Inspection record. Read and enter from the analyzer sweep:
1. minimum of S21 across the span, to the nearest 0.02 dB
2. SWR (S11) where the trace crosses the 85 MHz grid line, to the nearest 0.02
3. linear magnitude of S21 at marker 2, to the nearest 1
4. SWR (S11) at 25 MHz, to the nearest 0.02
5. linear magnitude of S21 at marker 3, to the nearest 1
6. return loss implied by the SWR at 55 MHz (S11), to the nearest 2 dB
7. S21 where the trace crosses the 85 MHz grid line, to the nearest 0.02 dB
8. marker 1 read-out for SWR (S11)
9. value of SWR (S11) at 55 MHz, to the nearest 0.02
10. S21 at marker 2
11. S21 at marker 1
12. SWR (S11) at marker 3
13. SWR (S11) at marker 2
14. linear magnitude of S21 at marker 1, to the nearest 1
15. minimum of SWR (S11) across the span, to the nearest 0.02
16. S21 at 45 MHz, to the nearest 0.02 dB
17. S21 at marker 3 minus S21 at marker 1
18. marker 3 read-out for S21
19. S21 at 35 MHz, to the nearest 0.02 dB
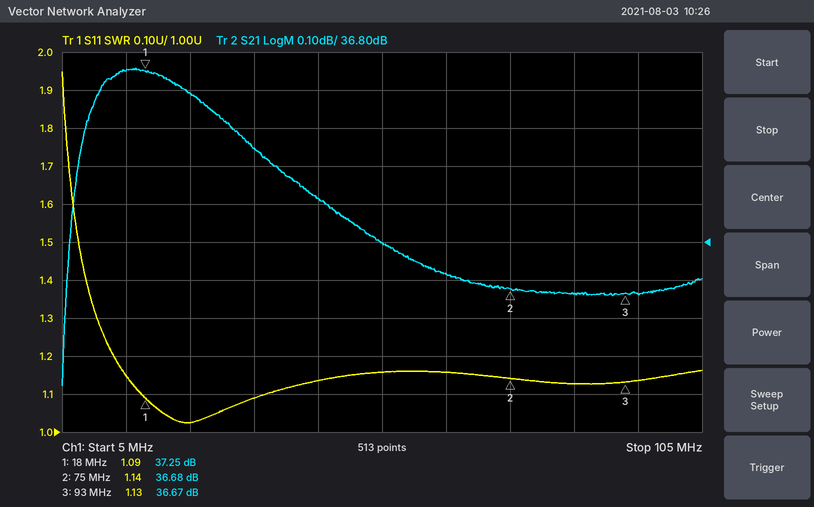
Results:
36.42 dB
1.12
68
1.02
68
22 dB
36.66 dB
1.09
1.16
36.68 dB
37.25 dB
1.13
1.14
73
1.02
36.92 dB
-0.58 dB
36.67 dB
37.04 dB
